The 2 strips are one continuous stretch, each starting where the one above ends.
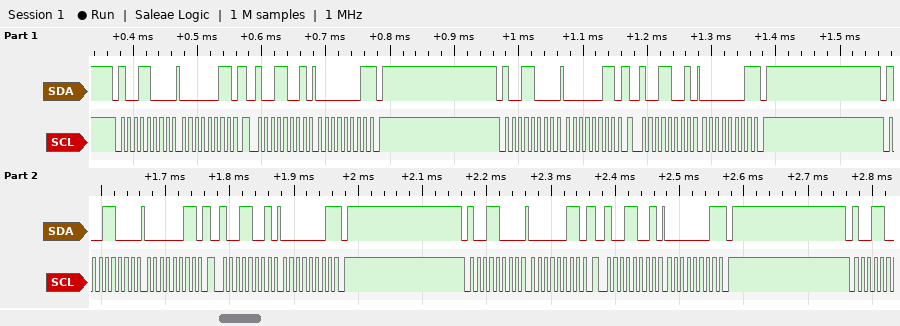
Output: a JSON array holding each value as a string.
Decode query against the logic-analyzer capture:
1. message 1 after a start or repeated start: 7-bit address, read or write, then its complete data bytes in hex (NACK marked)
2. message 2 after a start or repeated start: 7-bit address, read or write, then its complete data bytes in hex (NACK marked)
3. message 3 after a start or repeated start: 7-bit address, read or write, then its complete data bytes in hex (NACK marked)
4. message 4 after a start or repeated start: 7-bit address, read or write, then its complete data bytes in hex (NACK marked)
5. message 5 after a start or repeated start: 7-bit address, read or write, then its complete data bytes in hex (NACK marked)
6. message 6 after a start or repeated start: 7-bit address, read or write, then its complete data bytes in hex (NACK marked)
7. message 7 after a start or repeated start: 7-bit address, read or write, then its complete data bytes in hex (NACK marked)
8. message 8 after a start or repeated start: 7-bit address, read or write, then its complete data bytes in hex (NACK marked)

["0x4C write: 03", "0x4C read: 01 NACK", "0x4C write: 03", "0x4C read: 01 NACK", "0x4C write: 03", "0x4C read: 01 NACK", "0x4C write: 03", "0x4C read: 01 NACK"]
